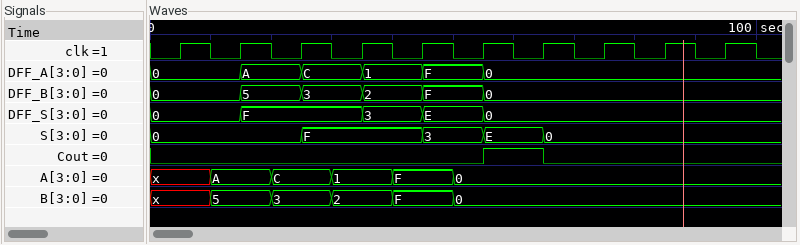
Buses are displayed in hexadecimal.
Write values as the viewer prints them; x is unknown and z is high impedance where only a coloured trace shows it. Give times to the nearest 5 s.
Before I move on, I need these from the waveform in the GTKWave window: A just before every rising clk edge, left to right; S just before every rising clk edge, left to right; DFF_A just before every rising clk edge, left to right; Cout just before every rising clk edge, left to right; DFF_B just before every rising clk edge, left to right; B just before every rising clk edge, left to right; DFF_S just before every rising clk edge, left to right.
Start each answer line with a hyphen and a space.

- x, A, C, 1, F, 0, 0, 0, 0, 0
- 0, 0, 0, F, F, 3, E, 0, 0, 0
- 0, 0, A, C, 1, F, 0, 0, 0, 0
- 0 0 0 0 0 0 1 0 0 0
- 0, 0, 5, 3, 2, F, 0, 0, 0, 0
- x, 5, 3, 2, F, 0, 0, 0, 0, 0
- 0, 0, F, F, 3, E, 0, 0, 0, 0
